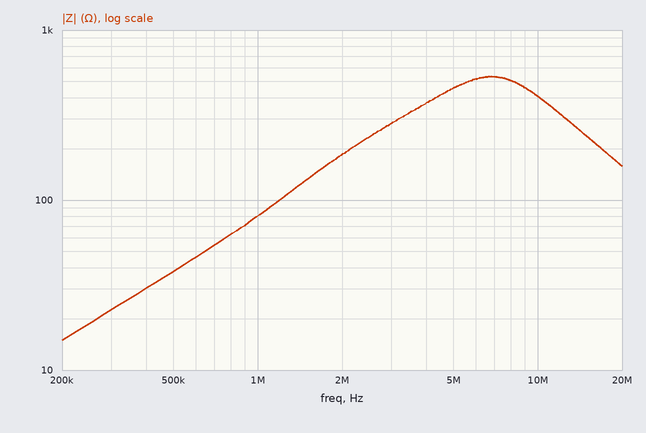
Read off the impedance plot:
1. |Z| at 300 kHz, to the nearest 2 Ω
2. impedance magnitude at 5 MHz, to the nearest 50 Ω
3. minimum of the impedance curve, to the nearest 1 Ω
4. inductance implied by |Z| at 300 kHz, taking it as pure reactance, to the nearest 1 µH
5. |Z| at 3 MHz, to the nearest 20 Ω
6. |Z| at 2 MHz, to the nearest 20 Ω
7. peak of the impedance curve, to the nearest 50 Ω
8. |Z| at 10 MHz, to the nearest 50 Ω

22 Ω
450 Ω
15 Ω
12 µH
280 Ω
180 Ω
550 Ω
400 Ω
